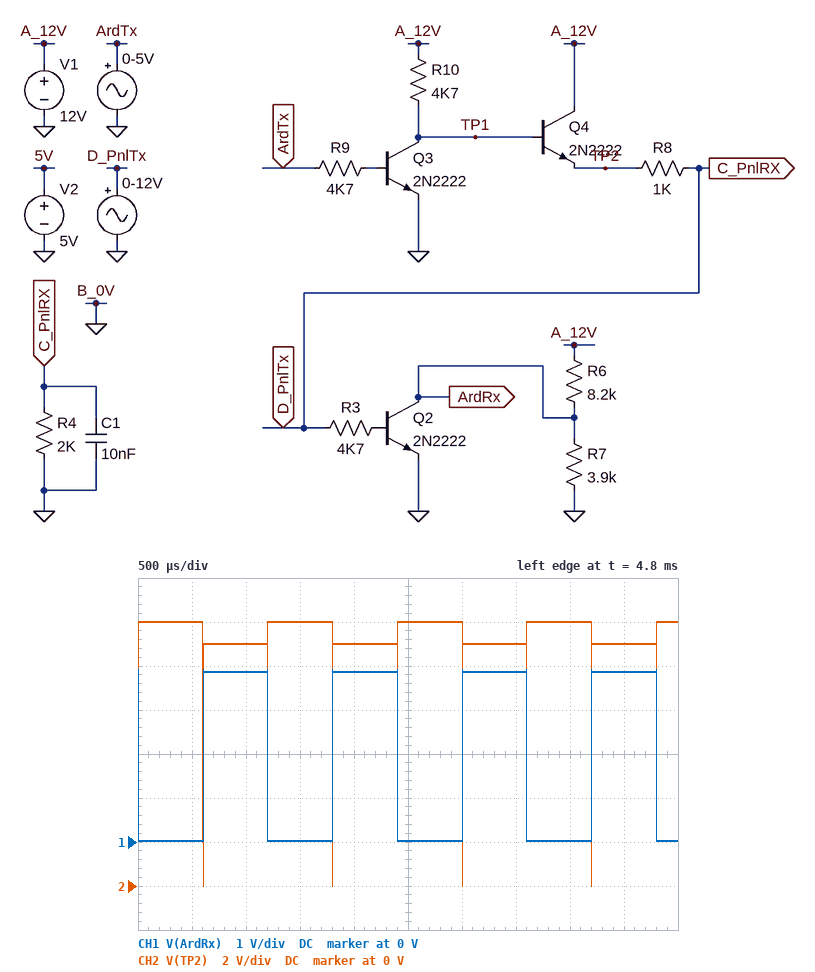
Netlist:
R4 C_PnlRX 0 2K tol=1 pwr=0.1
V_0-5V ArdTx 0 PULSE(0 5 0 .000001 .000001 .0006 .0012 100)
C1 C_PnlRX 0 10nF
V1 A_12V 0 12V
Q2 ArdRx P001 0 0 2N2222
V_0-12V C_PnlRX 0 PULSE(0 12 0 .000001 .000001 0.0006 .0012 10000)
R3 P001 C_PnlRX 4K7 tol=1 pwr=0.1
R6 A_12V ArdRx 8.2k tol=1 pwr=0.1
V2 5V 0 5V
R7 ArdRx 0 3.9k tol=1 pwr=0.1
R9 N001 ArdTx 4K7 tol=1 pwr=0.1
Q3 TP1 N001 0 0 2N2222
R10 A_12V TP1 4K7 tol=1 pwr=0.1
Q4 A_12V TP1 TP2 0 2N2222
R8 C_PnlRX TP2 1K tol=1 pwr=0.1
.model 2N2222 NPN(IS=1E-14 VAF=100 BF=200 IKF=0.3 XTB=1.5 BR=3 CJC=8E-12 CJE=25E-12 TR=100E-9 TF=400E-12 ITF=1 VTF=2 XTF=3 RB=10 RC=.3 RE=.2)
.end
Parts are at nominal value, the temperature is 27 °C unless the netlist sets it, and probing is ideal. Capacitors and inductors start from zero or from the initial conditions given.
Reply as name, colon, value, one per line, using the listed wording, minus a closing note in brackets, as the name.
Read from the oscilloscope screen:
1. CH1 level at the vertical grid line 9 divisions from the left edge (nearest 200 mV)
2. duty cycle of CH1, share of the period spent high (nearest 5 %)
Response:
CH1 level at the vertical grid line 9 divisions from the left edge: 3.8 V
duty cycle of CH1, share of the period spent high: 50 %
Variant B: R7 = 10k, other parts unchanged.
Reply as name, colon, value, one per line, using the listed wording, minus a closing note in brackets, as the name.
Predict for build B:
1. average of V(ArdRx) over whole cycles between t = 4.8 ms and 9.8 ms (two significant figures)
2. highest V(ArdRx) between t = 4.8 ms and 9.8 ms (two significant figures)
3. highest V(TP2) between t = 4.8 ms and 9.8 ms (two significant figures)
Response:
average of V(ArdRx) over whole cycles between t = 4.8 ms and 9.8 ms: 3.3 V
highest V(ArdRx) between t = 4.8 ms and 9.8 ms: 6.7 V
highest V(TP2) between t = 4.8 ms and 9.8 ms: 12 V
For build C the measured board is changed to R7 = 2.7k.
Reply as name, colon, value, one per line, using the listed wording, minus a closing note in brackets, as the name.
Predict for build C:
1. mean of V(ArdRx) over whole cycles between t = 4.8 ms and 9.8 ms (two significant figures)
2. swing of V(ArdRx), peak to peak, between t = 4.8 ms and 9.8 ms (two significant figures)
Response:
mean of V(ArdRx) over whole cycles between t = 4.8 ms and 9.8 ms: 1.5 V
swing of V(ArdRx), peak to peak, between t = 4.8 ms and 9.8 ms: 3.0 V
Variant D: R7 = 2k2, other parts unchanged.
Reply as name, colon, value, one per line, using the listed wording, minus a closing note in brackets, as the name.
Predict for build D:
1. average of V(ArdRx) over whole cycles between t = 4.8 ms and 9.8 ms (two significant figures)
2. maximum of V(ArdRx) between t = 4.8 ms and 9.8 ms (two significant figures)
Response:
average of V(ArdRx) over whole cycles between t = 4.8 ms and 9.8 ms: 1.3 V
maximum of V(ArdRx) between t = 4.8 ms and 9.8 ms: 2.6 V
